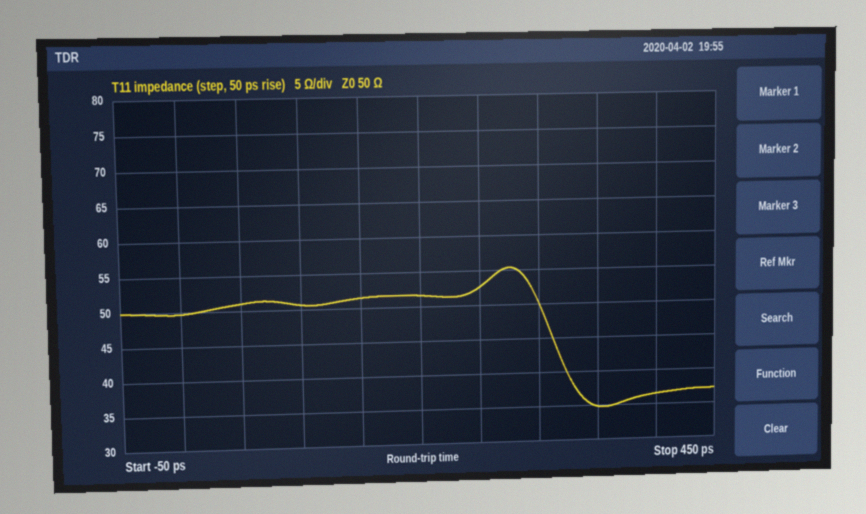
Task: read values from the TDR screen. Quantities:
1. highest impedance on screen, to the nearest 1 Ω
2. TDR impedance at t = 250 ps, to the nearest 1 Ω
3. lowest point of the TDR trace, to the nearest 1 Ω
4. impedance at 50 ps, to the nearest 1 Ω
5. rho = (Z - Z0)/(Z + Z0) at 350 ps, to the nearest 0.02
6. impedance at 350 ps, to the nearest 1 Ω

55 Ω
53 Ω
35 Ω
51 Ω
-0.18
35 Ω
